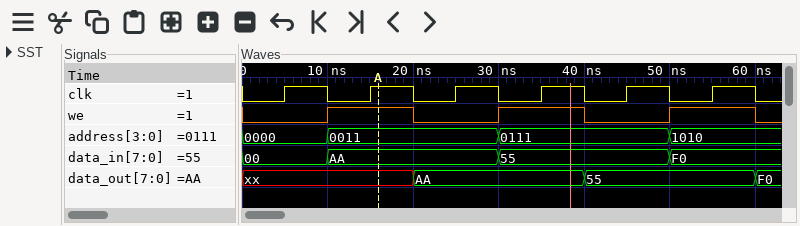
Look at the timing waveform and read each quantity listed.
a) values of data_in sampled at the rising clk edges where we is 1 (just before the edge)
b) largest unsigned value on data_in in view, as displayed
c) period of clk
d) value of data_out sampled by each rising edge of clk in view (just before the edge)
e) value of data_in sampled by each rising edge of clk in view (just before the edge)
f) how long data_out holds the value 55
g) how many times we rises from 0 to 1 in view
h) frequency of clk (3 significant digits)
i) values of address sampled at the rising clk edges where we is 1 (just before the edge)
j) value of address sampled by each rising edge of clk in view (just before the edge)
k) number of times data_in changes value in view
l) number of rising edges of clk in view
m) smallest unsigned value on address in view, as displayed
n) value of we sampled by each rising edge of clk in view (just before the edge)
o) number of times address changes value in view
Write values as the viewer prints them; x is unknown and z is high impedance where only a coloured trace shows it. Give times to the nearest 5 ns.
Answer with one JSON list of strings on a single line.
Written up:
["AA, 55, F0", "F0", "10 ns", "xx, xx, AA, AA, 55, 55", "00, AA, AA, 55, 55, F0", "20 ns", "3", "100 MHz", "0011, 0111, 1010", "0000, 0011, 0011, 0111, 0111, 1010", "3", "6", "0000", "0 1 0 1 0 1", "3"]
